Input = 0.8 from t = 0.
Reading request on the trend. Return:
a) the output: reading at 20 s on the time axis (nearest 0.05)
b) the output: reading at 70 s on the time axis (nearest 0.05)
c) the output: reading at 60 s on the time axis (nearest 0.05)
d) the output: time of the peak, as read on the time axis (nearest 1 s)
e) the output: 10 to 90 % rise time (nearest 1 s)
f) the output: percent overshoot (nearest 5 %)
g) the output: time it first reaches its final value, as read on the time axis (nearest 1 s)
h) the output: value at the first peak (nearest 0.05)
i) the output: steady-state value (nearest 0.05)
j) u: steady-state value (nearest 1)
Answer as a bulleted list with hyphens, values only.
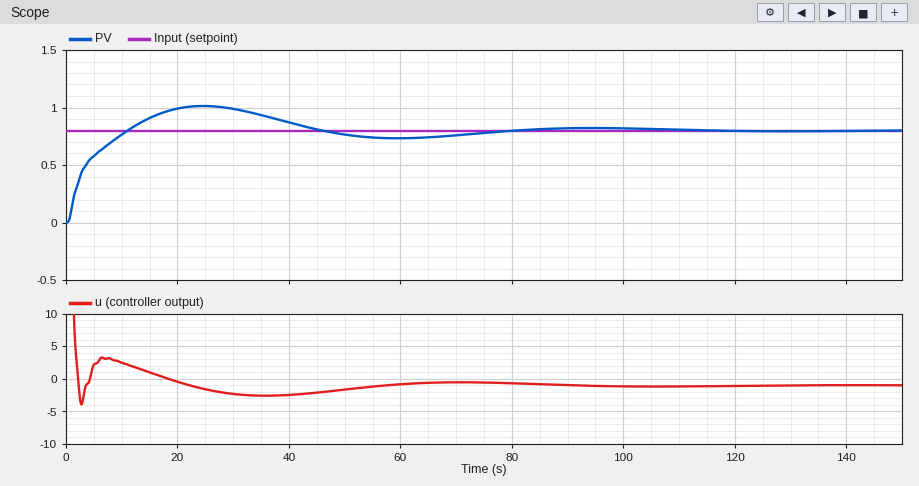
- 1.00
- 0.75
- 0.75
- 25 s
- 8 s
- 25 %
- 11 s
- 1.00
- 0.80
- -1
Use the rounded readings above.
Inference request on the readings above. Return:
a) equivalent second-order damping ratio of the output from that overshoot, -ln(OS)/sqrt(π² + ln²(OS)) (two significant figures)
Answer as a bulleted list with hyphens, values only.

- 0.40
